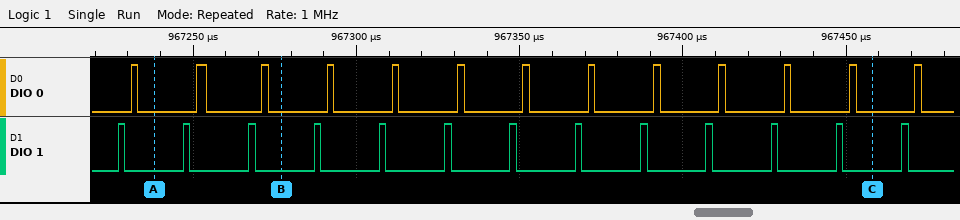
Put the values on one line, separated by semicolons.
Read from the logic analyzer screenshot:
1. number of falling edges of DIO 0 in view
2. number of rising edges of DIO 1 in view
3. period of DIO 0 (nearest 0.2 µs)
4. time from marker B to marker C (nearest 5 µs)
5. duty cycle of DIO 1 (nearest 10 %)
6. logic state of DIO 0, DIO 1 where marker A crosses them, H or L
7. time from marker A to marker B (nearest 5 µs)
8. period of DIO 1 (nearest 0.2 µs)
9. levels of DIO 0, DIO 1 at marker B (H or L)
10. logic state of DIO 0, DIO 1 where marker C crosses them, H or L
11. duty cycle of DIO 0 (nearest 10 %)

13; 13; 20 µs; 180 µs; 10 %; DIO 0=L, DIO 1=L; 40 µs; 20 µs; DIO 0=L, DIO 1=L; DIO 0=L, DIO 1=L; 10 %
